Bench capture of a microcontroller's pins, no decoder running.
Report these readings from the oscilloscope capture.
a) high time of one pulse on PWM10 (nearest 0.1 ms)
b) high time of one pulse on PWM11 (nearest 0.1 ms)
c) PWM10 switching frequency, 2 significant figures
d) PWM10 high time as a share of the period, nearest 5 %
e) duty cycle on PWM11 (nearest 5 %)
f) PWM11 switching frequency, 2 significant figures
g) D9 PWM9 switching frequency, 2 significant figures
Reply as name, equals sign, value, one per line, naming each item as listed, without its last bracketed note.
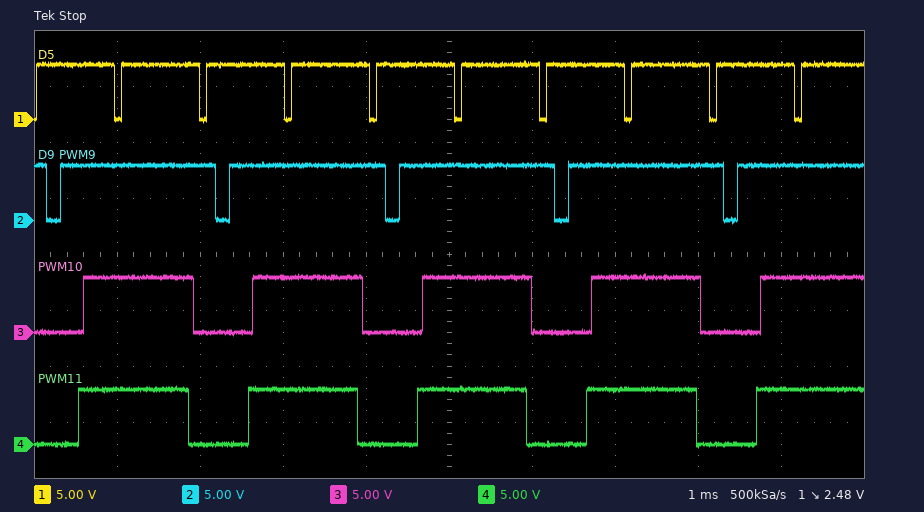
high time of one pulse on PWM10 = 1.3 ms
high time of one pulse on PWM11 = 1.3 ms
PWM10 switching frequency, 2 significant figures = 490 Hz
PWM10 high time as a share of the period, nearest 5 % = 65 %
duty cycle on PWM11 = 65 %
PWM11 switching frequency, 2 significant figures = 490 Hz
D9 PWM9 switching frequency, 2 significant figures = 490 Hz
